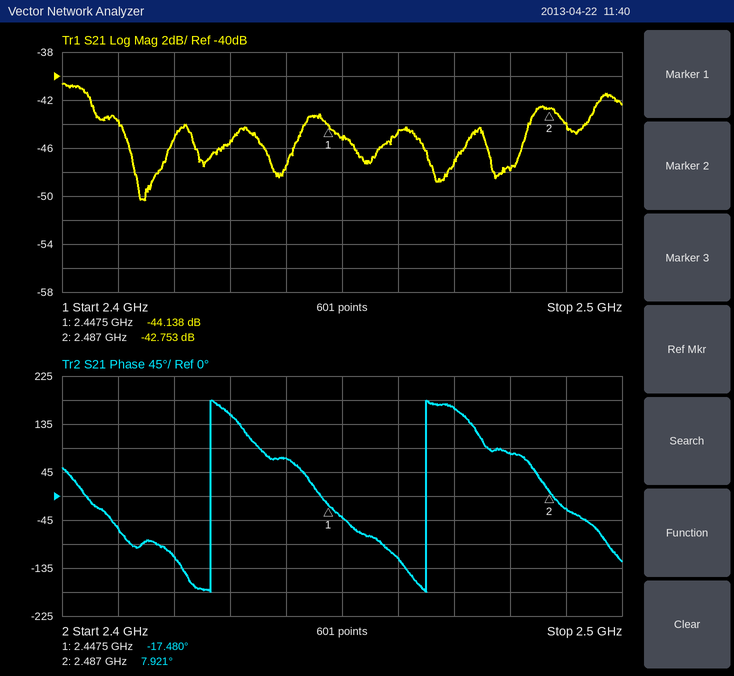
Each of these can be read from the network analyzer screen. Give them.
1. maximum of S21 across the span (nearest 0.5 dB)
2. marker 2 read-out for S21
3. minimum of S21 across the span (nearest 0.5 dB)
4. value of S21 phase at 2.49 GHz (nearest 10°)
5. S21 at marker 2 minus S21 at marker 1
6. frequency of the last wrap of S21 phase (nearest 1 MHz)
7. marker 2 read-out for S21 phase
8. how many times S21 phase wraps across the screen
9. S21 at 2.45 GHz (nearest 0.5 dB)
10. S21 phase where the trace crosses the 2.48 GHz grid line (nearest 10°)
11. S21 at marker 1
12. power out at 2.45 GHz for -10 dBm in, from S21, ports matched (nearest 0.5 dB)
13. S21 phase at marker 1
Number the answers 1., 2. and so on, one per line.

1. -40.5 dB
2. -42.753 dB
3. -50.5 dB
4. -20°
5. 1.385 dB
6. 2.465 GHz
7. 7.921°
8. 2
9. -45.0 dB
10. 80°
11. -44.138 dB
12. -55.0 dBm
13. -17.480°
